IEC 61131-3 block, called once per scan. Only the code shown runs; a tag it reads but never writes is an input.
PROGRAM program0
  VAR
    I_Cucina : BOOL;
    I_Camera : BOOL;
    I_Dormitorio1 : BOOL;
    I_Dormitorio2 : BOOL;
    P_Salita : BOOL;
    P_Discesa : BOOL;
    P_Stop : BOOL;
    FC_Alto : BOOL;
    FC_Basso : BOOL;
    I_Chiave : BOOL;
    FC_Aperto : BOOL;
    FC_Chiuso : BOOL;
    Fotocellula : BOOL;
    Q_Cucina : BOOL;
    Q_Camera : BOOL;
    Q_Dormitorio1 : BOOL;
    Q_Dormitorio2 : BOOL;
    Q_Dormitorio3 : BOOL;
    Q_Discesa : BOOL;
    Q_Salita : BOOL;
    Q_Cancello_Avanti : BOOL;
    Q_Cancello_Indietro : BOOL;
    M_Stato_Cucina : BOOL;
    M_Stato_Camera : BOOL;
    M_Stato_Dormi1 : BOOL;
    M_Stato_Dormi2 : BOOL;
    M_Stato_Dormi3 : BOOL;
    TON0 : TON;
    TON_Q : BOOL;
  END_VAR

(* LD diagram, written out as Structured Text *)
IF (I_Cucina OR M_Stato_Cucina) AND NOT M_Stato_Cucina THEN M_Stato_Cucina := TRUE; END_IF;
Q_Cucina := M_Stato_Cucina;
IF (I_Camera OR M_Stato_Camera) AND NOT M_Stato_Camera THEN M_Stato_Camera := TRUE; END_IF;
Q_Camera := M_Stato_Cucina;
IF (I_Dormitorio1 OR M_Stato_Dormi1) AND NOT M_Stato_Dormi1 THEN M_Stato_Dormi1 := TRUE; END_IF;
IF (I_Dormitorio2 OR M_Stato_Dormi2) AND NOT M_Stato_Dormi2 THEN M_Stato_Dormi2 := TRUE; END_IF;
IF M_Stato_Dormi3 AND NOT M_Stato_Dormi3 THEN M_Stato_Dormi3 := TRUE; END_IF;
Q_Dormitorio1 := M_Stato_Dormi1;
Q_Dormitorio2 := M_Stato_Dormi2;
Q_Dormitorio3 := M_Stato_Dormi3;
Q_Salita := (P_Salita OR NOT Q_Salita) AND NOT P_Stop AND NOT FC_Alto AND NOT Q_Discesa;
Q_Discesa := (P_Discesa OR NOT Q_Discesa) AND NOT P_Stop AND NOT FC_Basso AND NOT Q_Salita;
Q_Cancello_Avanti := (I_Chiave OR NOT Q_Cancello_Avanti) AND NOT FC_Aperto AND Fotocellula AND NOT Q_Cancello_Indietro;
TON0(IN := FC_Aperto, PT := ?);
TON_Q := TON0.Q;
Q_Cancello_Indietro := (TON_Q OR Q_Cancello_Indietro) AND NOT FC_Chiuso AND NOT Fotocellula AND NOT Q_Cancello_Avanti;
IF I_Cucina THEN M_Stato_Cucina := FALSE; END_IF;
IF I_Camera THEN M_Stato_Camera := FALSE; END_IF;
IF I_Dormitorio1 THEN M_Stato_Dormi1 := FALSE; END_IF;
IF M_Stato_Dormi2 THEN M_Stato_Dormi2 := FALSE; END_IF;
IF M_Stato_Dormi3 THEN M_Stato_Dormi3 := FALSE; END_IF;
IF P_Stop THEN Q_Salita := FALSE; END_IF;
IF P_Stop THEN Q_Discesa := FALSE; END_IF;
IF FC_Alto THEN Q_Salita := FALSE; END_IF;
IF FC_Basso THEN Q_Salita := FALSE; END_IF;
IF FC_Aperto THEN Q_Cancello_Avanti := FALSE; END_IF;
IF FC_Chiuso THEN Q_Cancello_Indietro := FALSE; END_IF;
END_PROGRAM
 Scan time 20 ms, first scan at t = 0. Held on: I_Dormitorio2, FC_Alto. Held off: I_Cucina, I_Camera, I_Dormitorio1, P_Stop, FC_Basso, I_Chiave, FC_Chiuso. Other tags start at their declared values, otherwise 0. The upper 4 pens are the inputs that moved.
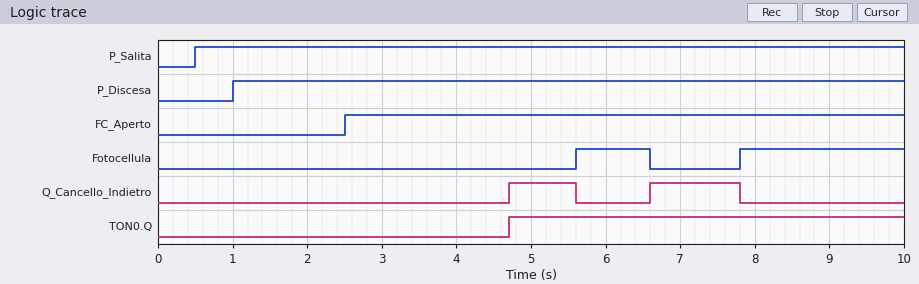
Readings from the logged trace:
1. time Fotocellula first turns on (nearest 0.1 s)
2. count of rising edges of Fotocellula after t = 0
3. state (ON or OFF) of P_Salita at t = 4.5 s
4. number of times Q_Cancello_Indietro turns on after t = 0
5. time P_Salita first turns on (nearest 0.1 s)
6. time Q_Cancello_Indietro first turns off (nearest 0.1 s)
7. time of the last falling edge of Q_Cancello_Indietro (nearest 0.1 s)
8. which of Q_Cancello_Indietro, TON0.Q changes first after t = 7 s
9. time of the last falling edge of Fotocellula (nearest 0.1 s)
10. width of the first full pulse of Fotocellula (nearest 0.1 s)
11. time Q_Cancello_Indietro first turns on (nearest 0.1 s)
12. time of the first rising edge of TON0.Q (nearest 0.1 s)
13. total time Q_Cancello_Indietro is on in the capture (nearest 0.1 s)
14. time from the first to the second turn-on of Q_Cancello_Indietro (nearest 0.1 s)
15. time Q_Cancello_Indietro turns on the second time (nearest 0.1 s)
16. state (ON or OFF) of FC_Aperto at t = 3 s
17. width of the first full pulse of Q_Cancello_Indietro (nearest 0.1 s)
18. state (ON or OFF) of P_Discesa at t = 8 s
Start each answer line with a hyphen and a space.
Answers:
- 5.6 s
- 2
- ON
- 2
- 0.5 s
- 5.6 s
- 7.8 s
- Q_Cancello_Indietro
- 6.6 s
- 1.0 s
- 4.7 s
- 4.7 s
- 2.1 s
- 1.9 s
- 6.6 s
- ON
- 0.9 s
- ON
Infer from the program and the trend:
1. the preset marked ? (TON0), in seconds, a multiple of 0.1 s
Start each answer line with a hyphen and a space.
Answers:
- 2.2 s
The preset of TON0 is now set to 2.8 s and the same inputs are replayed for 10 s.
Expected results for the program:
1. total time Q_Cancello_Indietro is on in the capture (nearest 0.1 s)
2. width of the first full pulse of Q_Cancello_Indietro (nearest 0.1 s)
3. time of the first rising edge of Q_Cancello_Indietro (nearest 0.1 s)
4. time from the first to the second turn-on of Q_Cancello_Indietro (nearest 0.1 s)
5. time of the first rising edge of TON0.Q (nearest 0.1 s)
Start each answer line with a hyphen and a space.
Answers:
- 1.5 s
- 0.3 s
- 5.3 s
- 1.3 s
- 5.3 s
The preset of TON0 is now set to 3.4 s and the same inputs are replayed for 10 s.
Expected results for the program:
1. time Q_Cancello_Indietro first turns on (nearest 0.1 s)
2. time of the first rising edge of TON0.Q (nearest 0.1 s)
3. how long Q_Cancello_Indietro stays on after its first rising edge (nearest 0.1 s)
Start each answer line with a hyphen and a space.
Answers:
- 6.6 s
- 5.9 s
- 1.2 s
